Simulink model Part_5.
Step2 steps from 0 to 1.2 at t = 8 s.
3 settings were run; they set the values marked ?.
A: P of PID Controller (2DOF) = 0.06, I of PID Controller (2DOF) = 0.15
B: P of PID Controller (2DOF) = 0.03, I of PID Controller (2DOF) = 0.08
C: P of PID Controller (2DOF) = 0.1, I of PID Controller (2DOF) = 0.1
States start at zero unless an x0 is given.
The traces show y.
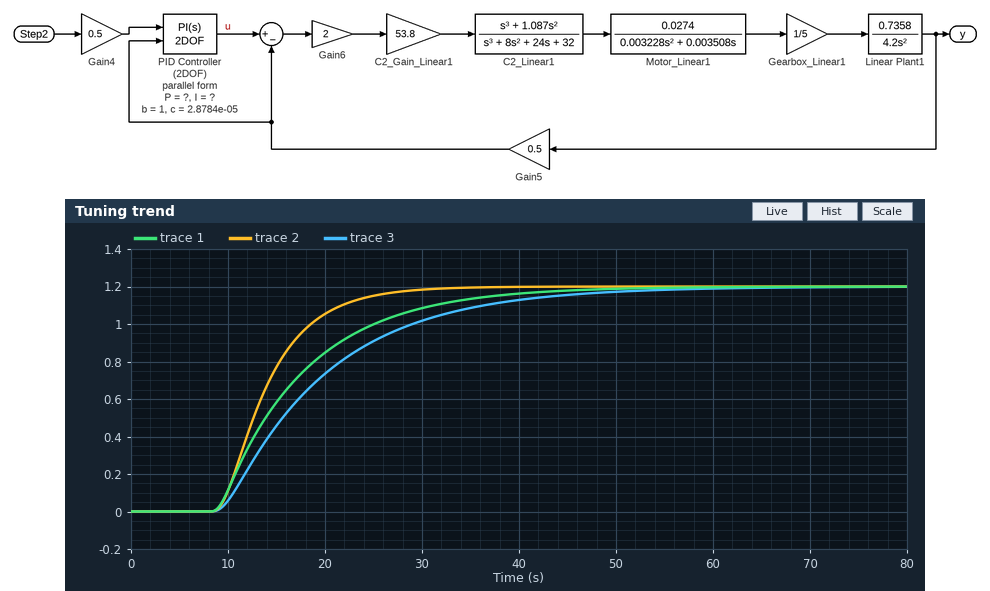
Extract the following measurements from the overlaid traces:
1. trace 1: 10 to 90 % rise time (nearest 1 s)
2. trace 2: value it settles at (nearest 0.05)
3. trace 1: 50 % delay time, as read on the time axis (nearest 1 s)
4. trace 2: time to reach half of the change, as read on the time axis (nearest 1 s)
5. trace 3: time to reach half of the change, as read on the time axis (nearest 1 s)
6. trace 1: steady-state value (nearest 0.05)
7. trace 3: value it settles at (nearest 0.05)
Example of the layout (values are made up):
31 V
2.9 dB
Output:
20 s
1.20
15 s
13 s
17 s
1.20
1.20
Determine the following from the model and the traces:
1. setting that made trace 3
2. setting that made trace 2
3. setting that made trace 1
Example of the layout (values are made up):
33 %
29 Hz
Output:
B
A
C
